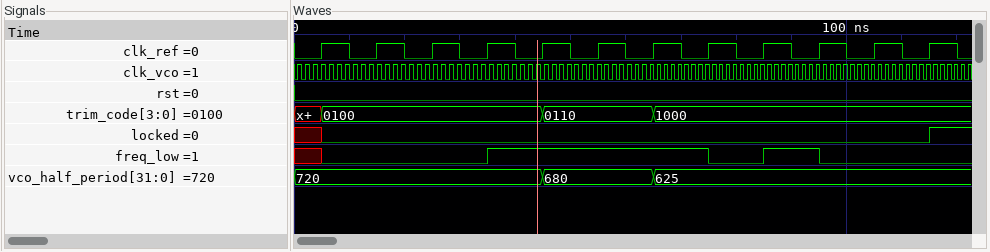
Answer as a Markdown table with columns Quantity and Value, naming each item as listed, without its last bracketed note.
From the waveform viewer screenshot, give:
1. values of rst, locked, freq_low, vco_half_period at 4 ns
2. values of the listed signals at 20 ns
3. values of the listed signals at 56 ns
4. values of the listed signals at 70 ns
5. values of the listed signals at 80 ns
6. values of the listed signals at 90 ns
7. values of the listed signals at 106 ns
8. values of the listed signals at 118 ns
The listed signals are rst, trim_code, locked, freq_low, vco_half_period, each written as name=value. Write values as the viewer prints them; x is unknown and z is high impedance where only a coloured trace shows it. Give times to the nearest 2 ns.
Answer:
| Quantity | Value |
|---|---|
| values of rst, locked, freq_low, vco_half_period at 4 ns | rst=0, locked=x, freq_low=x, vco_half_period=720 |
| values of the listed signals at 20 ns | rst=0, trim_code=0100, locked=0, freq_low=0, vco_half_period=720 |
| values of the listed signals at 56 ns | rst=0, trim_code=0110, locked=0, freq_low=1, vco_half_period=680 |
| values of the listed signals at 70 ns | rst=0, trim_code=1000, locked=0, freq_low=1, vco_half_period=625 |
| values of the listed signals at 80 ns | rst=0, trim_code=1000, locked=0, freq_low=0, vco_half_period=625 |
| values of the listed signals at 90 ns | rst=0, trim_code=1000, locked=0, freq_low=1, vco_half_period=625 |
| values of the listed signals at 106 ns | rst=0, trim_code=1000, locked=0, freq_low=0, vco_half_period=625 |
| values of the listed signals at 118 ns | rst=0, trim_code=1000, locked=1, freq_low=0, vco_half_period=625 |
